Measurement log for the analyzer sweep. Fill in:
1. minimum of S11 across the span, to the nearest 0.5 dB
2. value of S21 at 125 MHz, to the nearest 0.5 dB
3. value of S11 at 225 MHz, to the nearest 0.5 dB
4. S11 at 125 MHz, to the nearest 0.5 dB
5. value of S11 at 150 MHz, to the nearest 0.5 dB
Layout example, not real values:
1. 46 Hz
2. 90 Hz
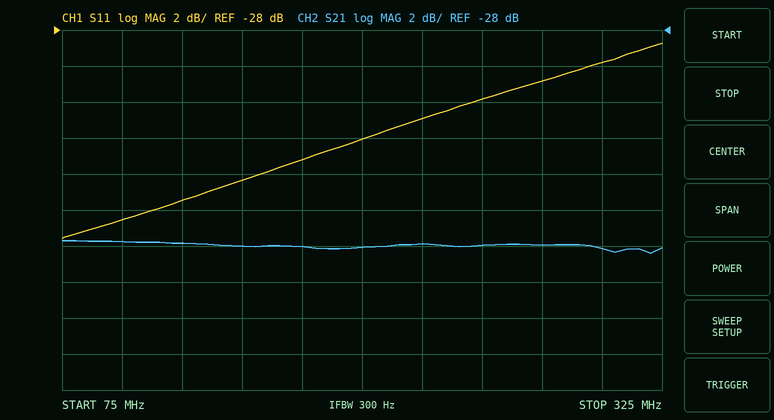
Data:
1. -39.5 dB
2. -40.0 dB
3. -33.0 dB
4. -37.5 dB
5. -36.5 dB
